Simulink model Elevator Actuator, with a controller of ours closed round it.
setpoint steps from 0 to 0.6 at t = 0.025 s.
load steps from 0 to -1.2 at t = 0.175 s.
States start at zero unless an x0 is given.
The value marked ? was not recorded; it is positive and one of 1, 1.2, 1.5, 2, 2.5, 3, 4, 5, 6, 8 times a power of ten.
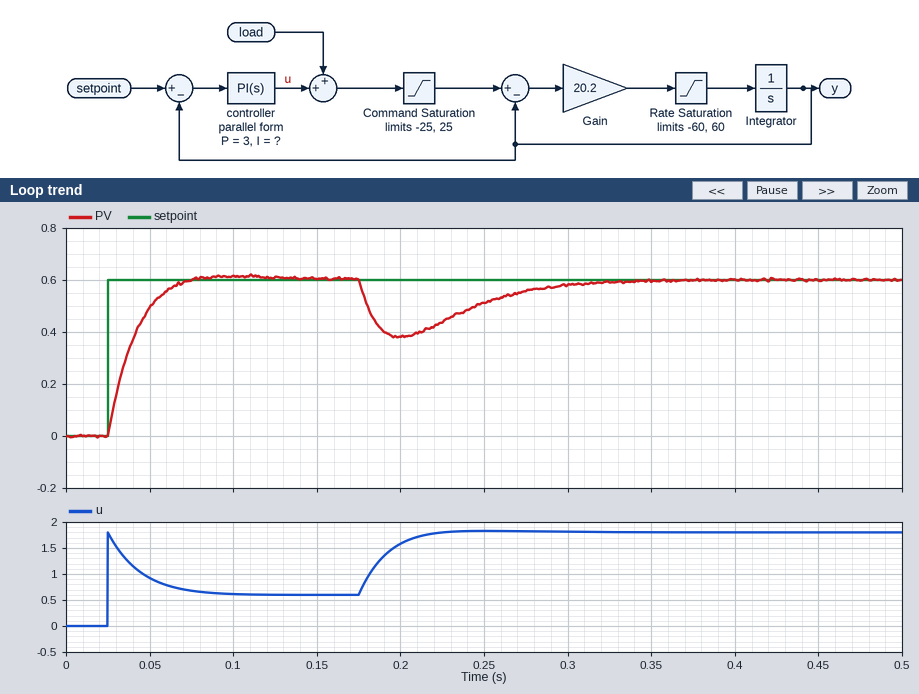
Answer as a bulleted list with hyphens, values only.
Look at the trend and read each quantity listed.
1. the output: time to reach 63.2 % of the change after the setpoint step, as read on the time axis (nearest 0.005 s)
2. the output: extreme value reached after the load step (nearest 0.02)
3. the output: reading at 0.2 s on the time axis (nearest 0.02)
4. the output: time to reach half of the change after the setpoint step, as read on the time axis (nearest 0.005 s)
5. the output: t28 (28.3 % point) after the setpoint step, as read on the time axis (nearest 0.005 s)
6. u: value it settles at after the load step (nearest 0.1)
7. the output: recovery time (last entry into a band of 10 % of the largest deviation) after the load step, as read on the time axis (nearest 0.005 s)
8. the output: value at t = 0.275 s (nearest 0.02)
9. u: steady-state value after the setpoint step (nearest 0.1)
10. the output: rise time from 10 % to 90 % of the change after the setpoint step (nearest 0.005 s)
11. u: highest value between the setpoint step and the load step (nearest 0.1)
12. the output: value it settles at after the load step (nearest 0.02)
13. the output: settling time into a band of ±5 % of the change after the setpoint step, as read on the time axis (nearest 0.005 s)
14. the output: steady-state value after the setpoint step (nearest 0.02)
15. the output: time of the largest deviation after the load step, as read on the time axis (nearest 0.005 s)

- 0.040 s
- 0.38
- 0.38
- 0.035 s
- 0.030 s
- 1.8
- 0.295 s
- 0.56
- 0.6
- 0.030 s
- 1.8
- 0.60
- 0.065 s
- 0.60
- 0.200 s
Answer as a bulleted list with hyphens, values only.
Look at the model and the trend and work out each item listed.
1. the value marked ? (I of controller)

- 80
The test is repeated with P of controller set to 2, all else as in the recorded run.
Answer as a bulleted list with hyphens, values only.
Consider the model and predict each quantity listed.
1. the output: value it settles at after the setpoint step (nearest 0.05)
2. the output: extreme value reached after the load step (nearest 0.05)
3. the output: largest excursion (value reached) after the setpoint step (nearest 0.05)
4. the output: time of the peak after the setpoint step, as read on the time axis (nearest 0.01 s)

- 0.60
- 0.35
- 0.65
- 0.10 s
